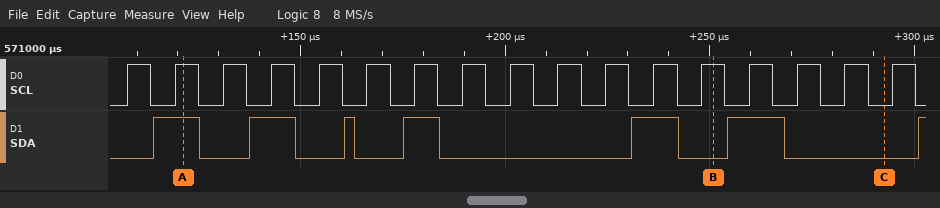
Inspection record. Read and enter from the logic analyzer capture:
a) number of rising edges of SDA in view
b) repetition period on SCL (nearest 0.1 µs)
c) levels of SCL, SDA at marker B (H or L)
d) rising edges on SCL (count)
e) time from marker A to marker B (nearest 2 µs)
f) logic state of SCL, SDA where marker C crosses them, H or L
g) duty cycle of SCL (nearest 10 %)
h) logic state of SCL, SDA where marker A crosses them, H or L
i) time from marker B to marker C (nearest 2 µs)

7
11.7 µs
SCL=H, SDA=L
17
130 µs
SCL=L, SDA=L
50 %
SCL=H, SDA=H
42 µs
